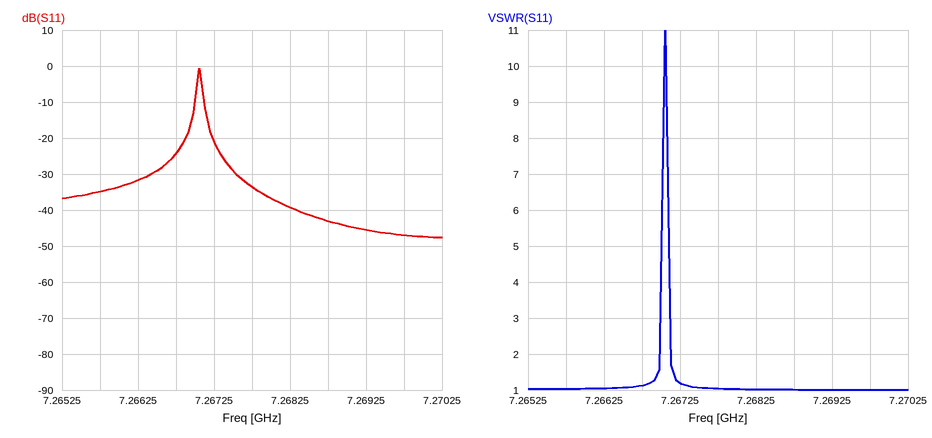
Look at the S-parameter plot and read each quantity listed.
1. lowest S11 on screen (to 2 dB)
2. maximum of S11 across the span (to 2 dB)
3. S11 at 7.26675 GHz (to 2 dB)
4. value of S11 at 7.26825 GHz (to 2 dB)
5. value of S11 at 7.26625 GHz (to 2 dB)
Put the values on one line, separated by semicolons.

-48 dB; 0 dB; -24 dB; -40 dB; -32 dB
